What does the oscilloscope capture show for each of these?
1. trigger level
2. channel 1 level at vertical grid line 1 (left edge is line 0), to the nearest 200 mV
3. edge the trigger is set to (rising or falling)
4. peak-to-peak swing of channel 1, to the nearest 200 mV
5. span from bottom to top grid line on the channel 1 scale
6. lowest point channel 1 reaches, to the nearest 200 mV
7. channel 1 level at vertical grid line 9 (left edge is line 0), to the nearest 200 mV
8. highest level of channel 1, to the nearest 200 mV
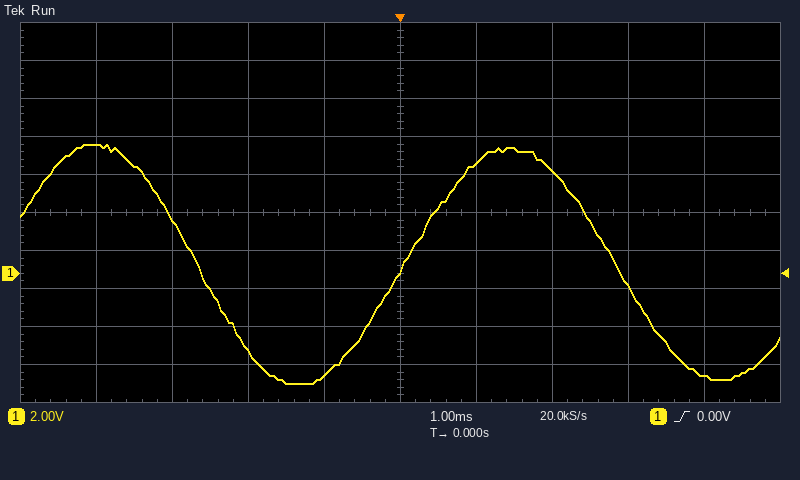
0.00 V
6.8 V
rising
12.6 V
20 V
-5.8 V
-5.4 V
6.8 V
